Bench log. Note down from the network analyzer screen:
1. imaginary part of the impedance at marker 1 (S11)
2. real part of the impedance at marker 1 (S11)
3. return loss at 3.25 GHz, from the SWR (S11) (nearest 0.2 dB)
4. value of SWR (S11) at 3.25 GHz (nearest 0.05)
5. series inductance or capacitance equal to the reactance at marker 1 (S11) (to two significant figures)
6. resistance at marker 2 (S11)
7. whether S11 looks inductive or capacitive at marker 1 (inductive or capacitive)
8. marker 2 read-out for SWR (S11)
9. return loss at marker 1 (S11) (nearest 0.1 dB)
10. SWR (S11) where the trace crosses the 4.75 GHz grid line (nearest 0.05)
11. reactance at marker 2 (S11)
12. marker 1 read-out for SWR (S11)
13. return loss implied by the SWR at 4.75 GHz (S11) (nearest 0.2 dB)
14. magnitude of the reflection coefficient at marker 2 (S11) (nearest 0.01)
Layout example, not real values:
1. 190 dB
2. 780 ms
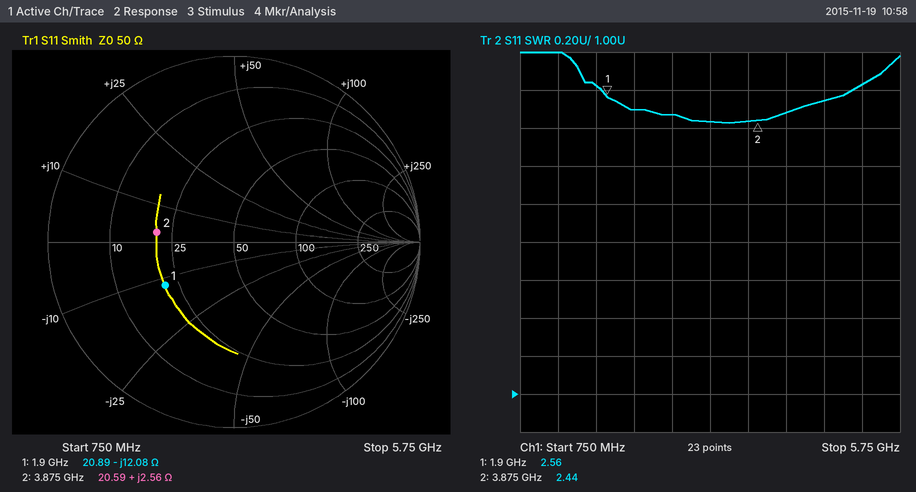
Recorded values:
1. -12.08 Ω
2. 20.89 Ω
3. 7.6 dB
4. 2.45
5. 6.9 pF
6. 20.59 Ω
7. capacitive
8. 2.44
9. 7.2 dB
10. 2.55
11. +2.56 Ω
12. 2.56
13. 7.2 dB
14. 0.42
